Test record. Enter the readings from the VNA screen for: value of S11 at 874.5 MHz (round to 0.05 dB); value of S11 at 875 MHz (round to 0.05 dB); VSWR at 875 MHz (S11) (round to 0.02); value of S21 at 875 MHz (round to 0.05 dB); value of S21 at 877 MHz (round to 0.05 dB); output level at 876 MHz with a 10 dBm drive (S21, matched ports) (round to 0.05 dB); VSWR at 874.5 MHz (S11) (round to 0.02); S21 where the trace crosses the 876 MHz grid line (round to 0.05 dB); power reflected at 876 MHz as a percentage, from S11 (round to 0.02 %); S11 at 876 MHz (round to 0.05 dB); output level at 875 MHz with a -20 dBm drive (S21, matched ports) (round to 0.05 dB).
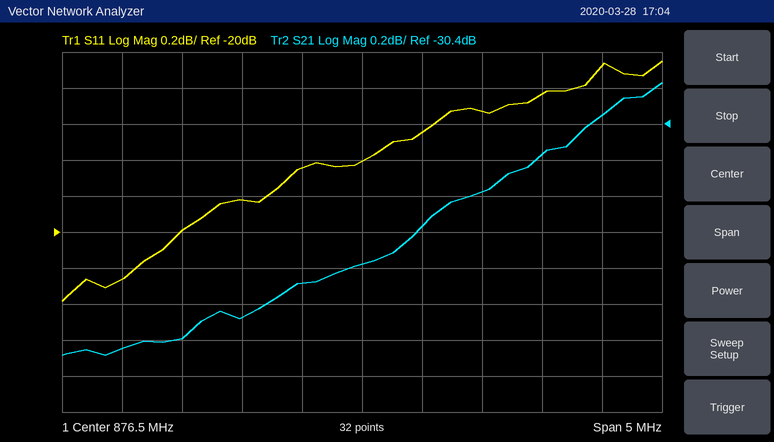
-20.25 dB
-20.00 dB
1.22
-31.60 dB
-30.95 dB
-21.30 dBm
1.22
-31.30 dB
1.08 %
-19.65 dB
-51.60 dBm
